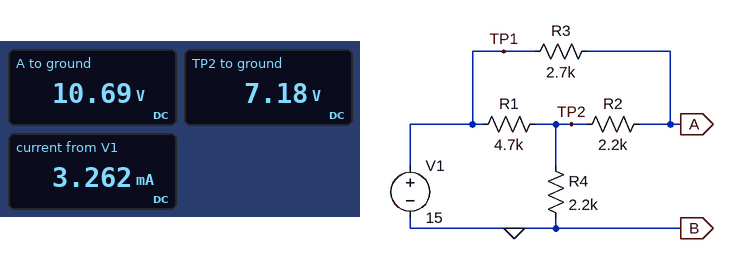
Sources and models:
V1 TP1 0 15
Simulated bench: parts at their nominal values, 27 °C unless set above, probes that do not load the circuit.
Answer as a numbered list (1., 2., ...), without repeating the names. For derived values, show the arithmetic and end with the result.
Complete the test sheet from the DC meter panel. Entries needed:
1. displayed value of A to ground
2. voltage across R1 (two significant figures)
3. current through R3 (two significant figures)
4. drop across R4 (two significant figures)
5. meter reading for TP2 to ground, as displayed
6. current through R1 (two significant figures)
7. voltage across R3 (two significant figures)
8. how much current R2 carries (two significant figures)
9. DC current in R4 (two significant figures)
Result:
1. 10.69 V
2. 15 V - 7.18 V = 7.8 V
3. (15 V - 10.69 V) / 2.7 kΩ = 1.6 mA
4. 7.18 V = 7.2 V
5. 7.18 V
6. (15 V - 7.18 V) / 4.7 kΩ = 1.7 mA
7. 15 V - 10.69 V = 4.3 V
8. (10.69 V - 7.18 V) / 2.2 kΩ = 1.6 mA
9. (7.18 V) / 2.2 kΩ = 3.3 mA
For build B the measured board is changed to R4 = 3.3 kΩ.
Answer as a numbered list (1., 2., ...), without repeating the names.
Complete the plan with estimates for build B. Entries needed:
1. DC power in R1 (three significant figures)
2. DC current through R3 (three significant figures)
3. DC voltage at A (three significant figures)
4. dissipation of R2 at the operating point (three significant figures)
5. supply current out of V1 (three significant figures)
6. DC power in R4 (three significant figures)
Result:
1. 8.48 mW
2. 1.29 mA
3. 11.5 V
4. 3.65 mW
5. 2.63 mA
6. 22.9 mW
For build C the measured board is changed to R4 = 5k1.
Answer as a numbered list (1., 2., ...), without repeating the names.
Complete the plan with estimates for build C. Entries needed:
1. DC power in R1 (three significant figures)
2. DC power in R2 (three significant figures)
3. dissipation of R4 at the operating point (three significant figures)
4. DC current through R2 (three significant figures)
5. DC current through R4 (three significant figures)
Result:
1. 4.90 mW
2. 2.11 mW
3. 20.4 mW
4. 979 µA
5. 2.00 mA
